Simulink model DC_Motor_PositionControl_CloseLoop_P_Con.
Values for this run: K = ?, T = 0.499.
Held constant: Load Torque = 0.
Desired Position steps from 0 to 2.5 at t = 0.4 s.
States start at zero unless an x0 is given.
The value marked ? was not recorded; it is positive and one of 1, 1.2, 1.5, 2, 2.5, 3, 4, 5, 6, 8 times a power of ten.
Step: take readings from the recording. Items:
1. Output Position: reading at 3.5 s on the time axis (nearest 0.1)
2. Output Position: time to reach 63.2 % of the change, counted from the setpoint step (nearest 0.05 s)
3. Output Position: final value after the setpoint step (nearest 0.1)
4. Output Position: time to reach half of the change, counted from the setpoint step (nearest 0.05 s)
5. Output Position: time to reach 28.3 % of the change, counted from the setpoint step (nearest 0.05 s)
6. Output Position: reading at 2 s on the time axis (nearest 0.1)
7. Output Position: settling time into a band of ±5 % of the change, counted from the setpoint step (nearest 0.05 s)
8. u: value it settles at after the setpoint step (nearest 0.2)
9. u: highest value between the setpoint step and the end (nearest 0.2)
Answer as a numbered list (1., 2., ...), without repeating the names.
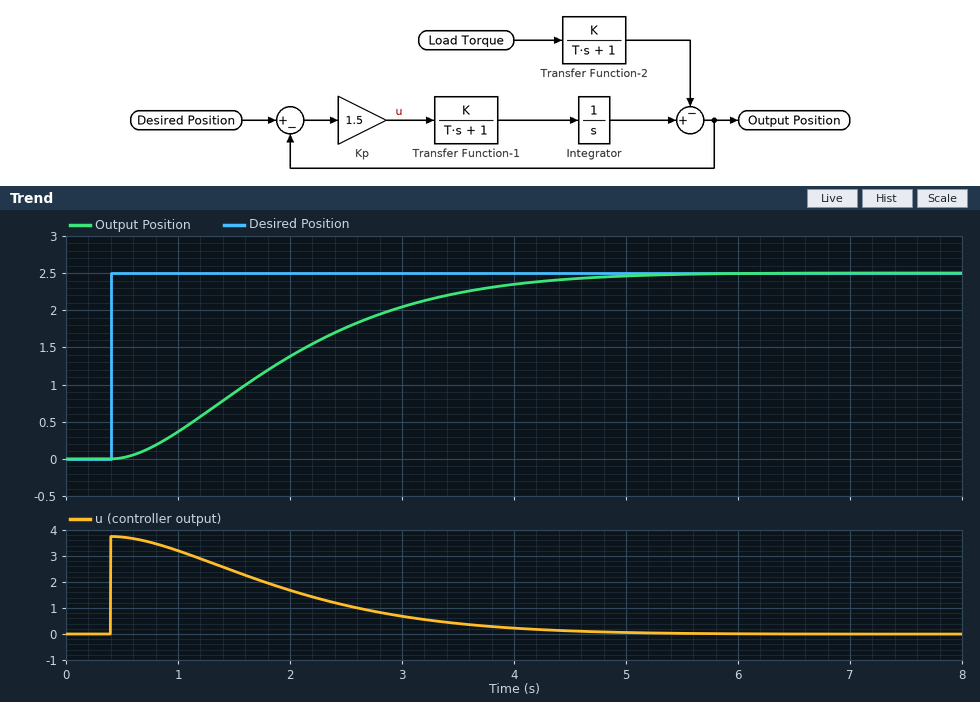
1. 2.2
2. 1.85 s
3. 2.5
4. 1.45 s
5. 0.95 s
6. 1.4
7. 3.75 s
8. 0.0
9. 3.8
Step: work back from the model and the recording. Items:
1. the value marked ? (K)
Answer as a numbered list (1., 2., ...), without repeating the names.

1. 0.4
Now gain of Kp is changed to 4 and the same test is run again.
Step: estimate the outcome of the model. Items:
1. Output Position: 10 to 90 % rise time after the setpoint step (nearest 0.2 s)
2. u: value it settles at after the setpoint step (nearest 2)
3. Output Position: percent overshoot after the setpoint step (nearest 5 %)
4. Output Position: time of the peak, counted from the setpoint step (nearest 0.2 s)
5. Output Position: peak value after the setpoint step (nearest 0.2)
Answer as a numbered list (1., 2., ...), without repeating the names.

1. 1.0 s
2. 0
3. 10 %
4. 2.2 s
5. 2.8
